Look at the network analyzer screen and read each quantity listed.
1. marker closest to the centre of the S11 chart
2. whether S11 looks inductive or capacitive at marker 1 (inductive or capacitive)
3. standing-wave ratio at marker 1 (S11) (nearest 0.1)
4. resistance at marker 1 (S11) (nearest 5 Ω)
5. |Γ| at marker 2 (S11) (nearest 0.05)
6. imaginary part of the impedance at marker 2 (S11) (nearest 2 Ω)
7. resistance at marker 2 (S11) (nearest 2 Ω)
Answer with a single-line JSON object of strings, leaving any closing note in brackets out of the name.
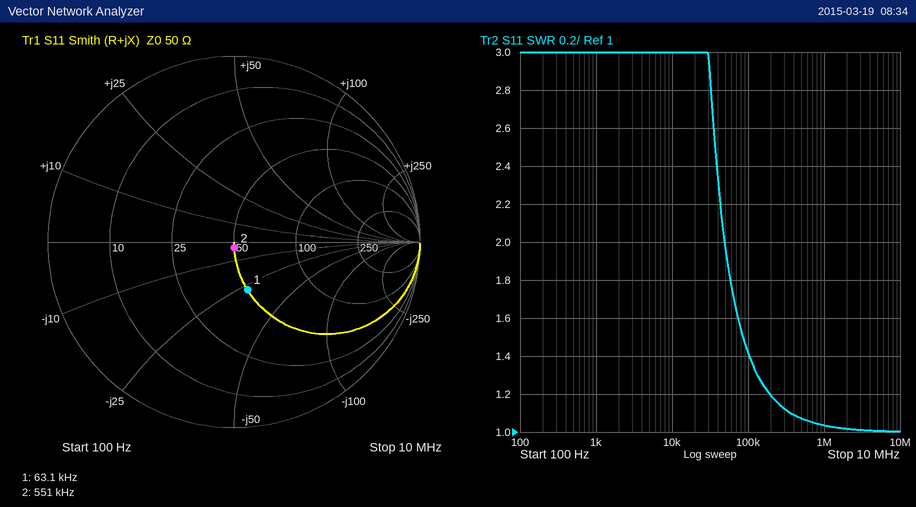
{"marker closest to the centre of the S11 chart": "marker 2", "whether S11 looks inductive or capacitive at marker 1": "capacitive", "standing-wave ratio at marker 1 (S11)": "1.7", "resistance at marker 1 (S11)": "50 Ω", "|Γ| at marker 2 (S11)": "0.05", "imaginary part of the impedance at marker 2 (S11)": "-4 Ω", "resistance at marker 2 (S11)": "50 Ω"}
